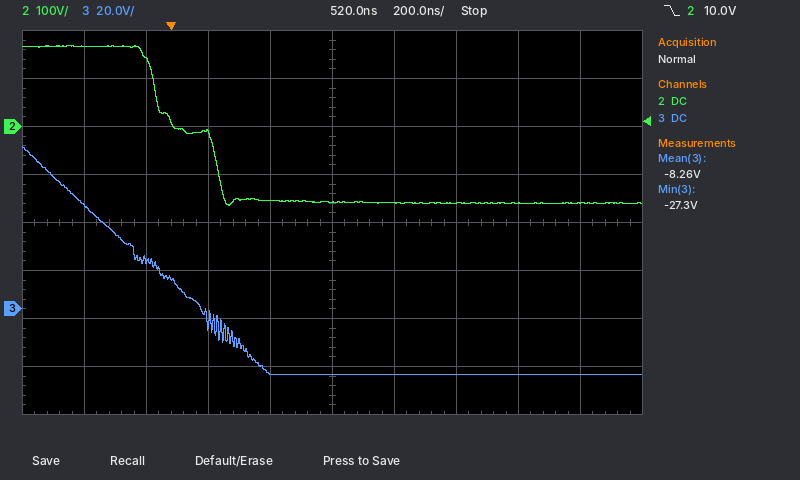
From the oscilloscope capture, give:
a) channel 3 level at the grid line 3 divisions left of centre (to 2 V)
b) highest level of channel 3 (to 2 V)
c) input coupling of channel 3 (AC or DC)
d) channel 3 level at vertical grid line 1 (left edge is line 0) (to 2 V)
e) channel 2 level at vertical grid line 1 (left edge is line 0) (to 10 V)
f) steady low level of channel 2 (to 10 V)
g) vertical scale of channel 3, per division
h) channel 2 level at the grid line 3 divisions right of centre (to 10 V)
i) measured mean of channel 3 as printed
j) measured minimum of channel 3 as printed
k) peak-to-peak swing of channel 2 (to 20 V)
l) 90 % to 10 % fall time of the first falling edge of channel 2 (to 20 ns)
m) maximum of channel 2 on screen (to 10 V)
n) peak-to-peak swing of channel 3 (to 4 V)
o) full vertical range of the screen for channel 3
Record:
20 V
68 V
DC
44 V
170 V
-160 V
20 V
-160 V
-8.26 V
-27.3 V
340 V
240 ns
170 V
96 V
160 V
